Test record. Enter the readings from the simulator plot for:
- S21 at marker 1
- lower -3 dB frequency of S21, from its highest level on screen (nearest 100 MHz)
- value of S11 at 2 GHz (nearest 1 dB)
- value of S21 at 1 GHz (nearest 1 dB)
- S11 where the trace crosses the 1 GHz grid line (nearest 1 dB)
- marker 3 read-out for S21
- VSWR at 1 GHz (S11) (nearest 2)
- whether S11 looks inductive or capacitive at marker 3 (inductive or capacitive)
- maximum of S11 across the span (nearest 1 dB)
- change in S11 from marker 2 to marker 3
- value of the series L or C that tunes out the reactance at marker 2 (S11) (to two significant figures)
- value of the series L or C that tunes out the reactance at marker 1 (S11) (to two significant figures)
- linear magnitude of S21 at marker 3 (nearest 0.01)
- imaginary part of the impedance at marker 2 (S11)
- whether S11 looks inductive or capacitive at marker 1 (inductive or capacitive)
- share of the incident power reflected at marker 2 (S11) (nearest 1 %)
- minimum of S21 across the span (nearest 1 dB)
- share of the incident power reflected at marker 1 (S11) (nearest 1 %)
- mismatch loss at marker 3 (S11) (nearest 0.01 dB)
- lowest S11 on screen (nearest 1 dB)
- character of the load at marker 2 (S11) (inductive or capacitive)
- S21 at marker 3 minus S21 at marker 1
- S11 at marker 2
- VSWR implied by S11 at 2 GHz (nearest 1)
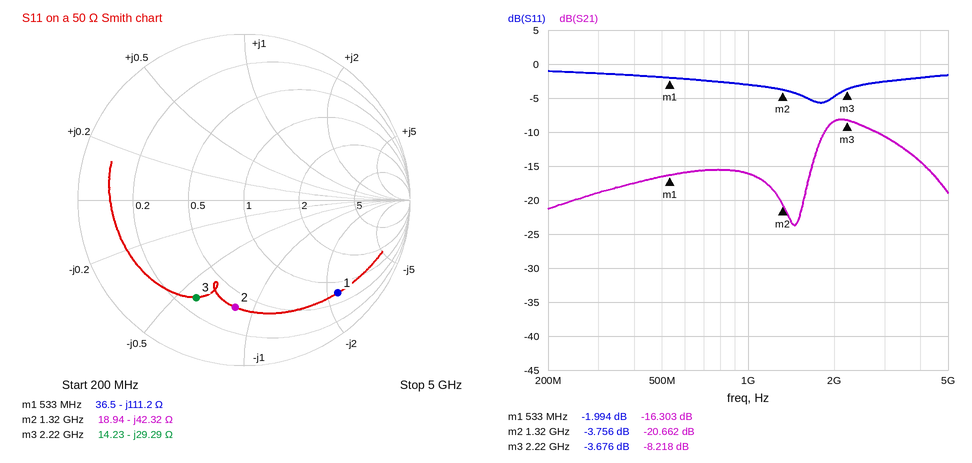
-16.303 dB
1.8 GHz
-5 dB
-16 dB
-3 dB
-8.218 dB
6
capacitive
-1 dB
0.080 dB
5.1 nH
33 nH
0.39
-42.32 Ω
capacitive
42 %
-24 dB
63 %
2.43 dB
-6 dB
capacitive
8.085 dB
-3.756 dB
4
